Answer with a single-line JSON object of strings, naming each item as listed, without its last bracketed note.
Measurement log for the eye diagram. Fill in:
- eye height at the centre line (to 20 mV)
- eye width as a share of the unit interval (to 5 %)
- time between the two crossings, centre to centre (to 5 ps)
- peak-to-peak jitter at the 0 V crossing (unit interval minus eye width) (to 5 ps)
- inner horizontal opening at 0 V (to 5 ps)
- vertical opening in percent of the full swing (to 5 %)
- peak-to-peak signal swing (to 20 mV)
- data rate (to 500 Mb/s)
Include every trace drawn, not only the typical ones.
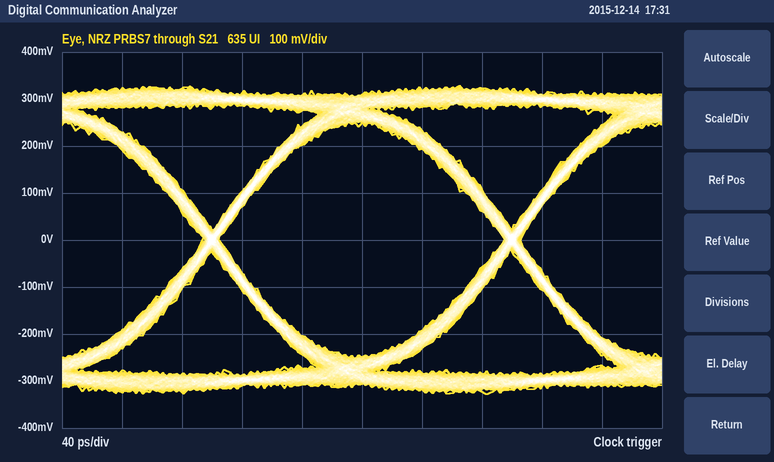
{"eye height at the centre line": "500 mV", "eye width as a share of the unit interval": "95 %", "time between the two crossings, centre to centre": "200 ps", "peak-to-peak jitter at the 0 V crossing (unit interval minus eye width)": "10 ps", "inner horizontal opening at 0 V": "190 ps", "vertical opening in percent of the full swing": "75 %", "peak-to-peak signal swing": "660 mV", "data rate": "5.0 Gb/s"}
